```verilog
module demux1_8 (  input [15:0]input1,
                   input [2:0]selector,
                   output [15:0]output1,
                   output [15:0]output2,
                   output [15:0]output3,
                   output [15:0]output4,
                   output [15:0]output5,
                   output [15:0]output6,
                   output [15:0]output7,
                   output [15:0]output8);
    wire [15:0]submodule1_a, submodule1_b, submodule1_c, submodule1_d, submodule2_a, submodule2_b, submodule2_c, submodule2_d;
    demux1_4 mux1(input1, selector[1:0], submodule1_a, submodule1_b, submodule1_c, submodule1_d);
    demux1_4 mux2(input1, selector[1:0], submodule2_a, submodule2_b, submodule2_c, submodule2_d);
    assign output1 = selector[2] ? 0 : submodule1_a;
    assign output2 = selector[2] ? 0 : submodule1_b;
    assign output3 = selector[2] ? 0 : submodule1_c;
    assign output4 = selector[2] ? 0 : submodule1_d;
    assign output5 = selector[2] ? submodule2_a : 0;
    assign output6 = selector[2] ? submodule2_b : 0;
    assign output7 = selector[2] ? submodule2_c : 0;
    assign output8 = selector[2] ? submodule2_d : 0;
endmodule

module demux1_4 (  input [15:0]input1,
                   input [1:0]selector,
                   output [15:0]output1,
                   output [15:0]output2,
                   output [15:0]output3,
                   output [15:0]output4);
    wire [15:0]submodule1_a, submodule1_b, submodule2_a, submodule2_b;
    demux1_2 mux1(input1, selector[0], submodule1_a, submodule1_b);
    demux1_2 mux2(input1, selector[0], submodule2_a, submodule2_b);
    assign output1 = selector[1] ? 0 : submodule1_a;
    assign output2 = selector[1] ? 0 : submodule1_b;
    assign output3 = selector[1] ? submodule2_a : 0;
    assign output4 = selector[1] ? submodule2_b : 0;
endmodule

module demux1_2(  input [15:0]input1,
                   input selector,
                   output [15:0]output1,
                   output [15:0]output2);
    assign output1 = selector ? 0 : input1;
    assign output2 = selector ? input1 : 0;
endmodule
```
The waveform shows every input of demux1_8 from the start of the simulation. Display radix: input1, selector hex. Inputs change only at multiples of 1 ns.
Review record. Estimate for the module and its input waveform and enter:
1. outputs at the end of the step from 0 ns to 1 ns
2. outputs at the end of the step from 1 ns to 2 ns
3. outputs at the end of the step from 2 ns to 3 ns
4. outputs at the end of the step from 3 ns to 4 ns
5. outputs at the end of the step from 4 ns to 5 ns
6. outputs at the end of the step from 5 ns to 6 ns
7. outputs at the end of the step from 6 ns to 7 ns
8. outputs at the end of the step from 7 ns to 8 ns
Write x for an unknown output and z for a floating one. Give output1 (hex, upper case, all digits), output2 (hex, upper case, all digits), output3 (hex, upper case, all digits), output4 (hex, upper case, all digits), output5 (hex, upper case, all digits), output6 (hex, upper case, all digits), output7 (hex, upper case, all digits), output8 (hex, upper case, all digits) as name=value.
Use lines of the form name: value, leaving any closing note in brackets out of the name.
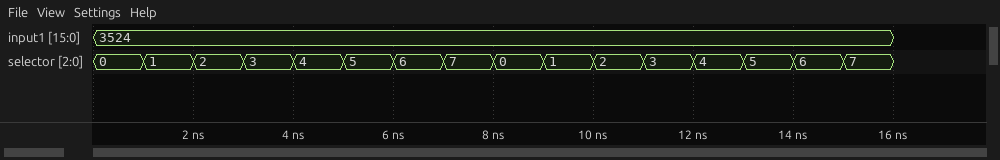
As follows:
outputs at the end of the step from 0 ns to 1 ns: output1=3524, output2=0000, output3=0000, output4=0000, output5=0000, output6=0000, output7=0000, output8=0000
outputs at the end of the step from 1 ns to 2 ns: output1=0000, output2=3524, output3=0000, output4=0000, output5=0000, output6=0000, output7=0000, output8=0000
outputs at the end of the step from 2 ns to 3 ns: output1=0000, output2=0000, output3=3524, output4=0000, output5=0000, output6=0000, output7=0000, output8=0000
outputs at the end of the step from 3 ns to 4 ns: output1=0000, output2=0000, output3=0000, output4=3524, output5=0000, output6=0000, output7=0000, output8=0000
outputs at the end of the step from 4 ns to 5 ns: output1=0000, output2=0000, output3=0000, output4=0000, output5=3524, output6=0000, output7=0000, output8=0000
outputs at the end of the step from 5 ns to 6 ns: output1=0000, output2=0000, output3=0000, output4=0000, output5=0000, output6=3524, output7=0000, output8=0000
outputs at the end of the step from 6 ns to 7 ns: output1=0000, output2=0000, output3=0000, output4=0000, output5=0000, output6=0000, output7=3524, output8=0000
outputs at the end of the step from 7 ns to 8 ns: output1=0000, output2=0000, output3=0000, output4=0000, output5=0000, output6=0000, output7=0000, output8=3524
